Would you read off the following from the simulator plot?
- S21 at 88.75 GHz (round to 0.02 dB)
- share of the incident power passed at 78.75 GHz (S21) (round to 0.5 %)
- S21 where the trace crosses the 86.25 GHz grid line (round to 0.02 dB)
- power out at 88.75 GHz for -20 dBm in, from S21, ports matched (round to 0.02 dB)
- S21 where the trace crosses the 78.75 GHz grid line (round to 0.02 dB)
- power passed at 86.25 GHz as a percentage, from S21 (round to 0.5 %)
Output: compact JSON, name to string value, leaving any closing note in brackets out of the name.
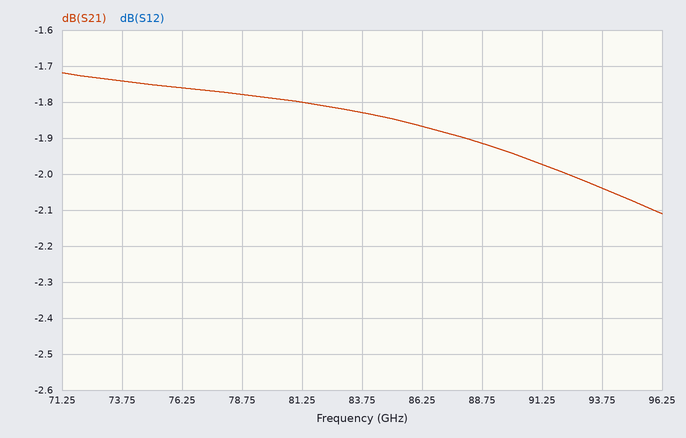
{"S21 at 88.75 GHz": "-1.92 dB", "share of the incident power passed at 78.75 GHz (S21)": "66.5 %", "S21 where the trace crosses the 86.25 GHz grid line": "-1.86 dB", "power out at 88.75 GHz for -20 dBm in, from S21, ports matched": "-21.92 dBm", "S21 where the trace crosses the 78.75 GHz grid line": "-1.78 dB", "power passed at 86.25 GHz as a percentage, from S21": "65.0 %"}
